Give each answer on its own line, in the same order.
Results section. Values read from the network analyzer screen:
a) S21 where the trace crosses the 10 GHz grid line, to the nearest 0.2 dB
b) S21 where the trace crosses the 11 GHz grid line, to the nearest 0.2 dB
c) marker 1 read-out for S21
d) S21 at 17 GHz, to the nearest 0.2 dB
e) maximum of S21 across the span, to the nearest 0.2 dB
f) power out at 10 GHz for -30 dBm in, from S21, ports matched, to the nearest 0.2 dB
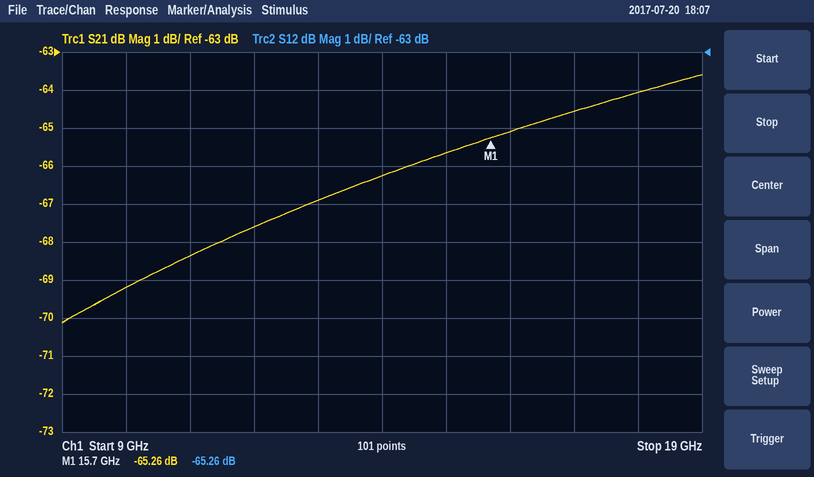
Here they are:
-69.2 dB
-68.4 dB
-65.26 dB
-64.6 dB
-63.6 dB
-99.2 dBm
